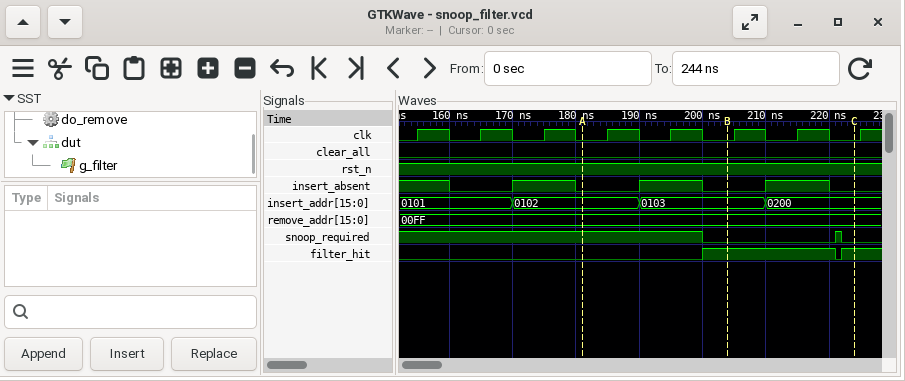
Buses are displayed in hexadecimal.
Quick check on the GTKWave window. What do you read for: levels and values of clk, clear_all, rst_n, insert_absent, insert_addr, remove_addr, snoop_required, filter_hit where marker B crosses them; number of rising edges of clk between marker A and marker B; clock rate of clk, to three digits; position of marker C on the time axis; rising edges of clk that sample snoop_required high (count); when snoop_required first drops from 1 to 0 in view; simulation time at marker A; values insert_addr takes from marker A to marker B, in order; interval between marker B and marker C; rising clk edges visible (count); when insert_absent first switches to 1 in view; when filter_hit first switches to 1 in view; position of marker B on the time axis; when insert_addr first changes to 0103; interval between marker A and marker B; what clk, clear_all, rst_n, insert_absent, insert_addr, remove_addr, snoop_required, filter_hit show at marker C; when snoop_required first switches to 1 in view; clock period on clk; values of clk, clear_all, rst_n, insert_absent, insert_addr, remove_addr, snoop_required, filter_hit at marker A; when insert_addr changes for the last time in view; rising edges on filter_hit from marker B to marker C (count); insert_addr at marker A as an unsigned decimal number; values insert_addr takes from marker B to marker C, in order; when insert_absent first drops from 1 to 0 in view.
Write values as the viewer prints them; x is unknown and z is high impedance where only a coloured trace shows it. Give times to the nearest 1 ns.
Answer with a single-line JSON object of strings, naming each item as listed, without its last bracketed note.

{"levels and values of clk, clear_all, rst_n, insert_absent, insert_addr, remove_addr, snoop_required, filter_hit where marker B crosses them": "clk=0, clear_all=0, rst_n=1, insert_absent=0, insert_addr=0103, remove_addr=00FF, snoop_required=0, filter_hit=1", "number of rising edges of clk between marker A and marker B": "2", "clock rate of clk, to three digits": "100 MHz", "position of marker C on the time axis": "224 ns", "rising edges of clk that sample snoop_required high": "5", "when snoop_required first drops from 1 to 0 in view": "200 ns", "simulation time at marker A": "181 ns", "values insert_addr takes from marker A to marker B, in order": "0102, 0103", "interval between marker B and marker C": "20 ns", "rising clk edges visible": "8", "when insert_absent first switches to 1 in view": "170 ns", "when filter_hit first switches to 1 in view": "200 ns", "position of marker B on the time axis": "204 ns", "when insert_addr first changes to 0103": "190 ns", "interval between marker A and marker B": "23 ns", "what clk, clear_all, rst_n, insert_absent, insert_addr, remove_addr, snoop_required, filter_hit show at marker C": "clk=0, clear_all=0, rst_n=1, insert_absent=0, insert_addr=0200, remove_addr=00FF, snoop_required=0, filter_hit=1", "when snoop_required first switches to 1 in view": "221 ns", "clock period on clk": "10 ns", "values of clk, clear_all, rst_n, insert_absent, insert_addr, remove_addr, snoop_required, filter_hit at marker A": "clk=0, clear_all=0, rst_n=1, insert_absent=0, insert_addr=0102, remove_addr=00FF, snoop_required=1, filter_hit=0", "when insert_addr changes for the last time in view": "210 ns", "rising edges on filter_hit from marker B to marker C": "1", "insert_addr at marker A as an unsigned decimal number": "258", "values insert_addr takes from marker B to marker C, in order": "0103, 0200", "when insert_absent first drops from 1 to 0 in view": "160 ns"}
